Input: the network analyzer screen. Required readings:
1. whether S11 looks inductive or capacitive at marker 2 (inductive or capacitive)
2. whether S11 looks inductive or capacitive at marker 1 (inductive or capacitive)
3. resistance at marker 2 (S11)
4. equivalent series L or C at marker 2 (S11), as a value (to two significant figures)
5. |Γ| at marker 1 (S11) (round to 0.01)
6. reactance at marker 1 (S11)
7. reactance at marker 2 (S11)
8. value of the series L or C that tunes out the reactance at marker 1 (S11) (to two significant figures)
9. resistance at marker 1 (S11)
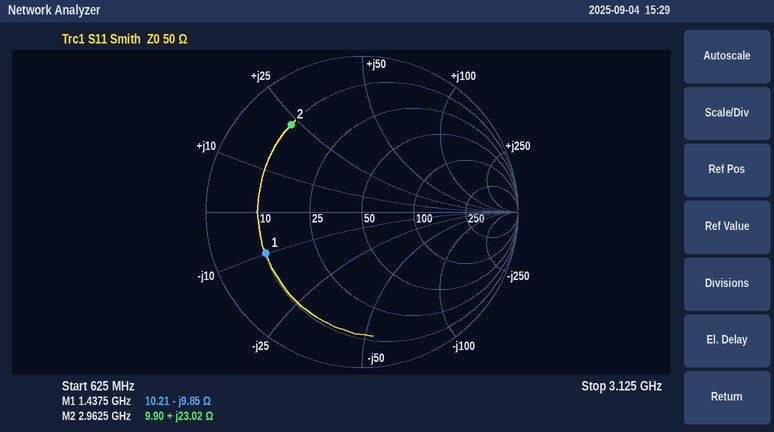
inductive
capacitive
9.90 Ω
1.2 nH
0.67
-9.85 Ω
+23.02 Ω
1.1 nH
10.21 Ω
